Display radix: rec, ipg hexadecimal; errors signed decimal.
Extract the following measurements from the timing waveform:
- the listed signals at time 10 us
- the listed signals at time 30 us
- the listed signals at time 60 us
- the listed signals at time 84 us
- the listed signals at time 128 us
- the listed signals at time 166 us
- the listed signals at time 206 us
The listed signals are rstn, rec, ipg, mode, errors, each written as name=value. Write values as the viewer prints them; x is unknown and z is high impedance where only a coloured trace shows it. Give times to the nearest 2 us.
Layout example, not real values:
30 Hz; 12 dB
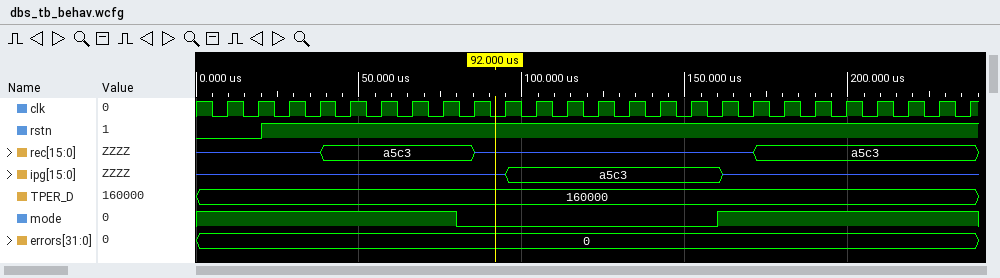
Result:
rstn=0, rec=z, ipg=z, mode=1, errors=0; rstn=1, rec=z, ipg=z, mode=1, errors=0; rstn=1, rec=a5c3, ipg=z, mode=1, errors=0; rstn=1, rec=a5c3, ipg=z, mode=0, errors=0; rstn=1, rec=z, ipg=a5c3, mode=0, errors=0; rstn=1, rec=z, ipg=z, mode=1, errors=0; rstn=1, rec=a5c3, ipg=z, mode=1, errors=0
